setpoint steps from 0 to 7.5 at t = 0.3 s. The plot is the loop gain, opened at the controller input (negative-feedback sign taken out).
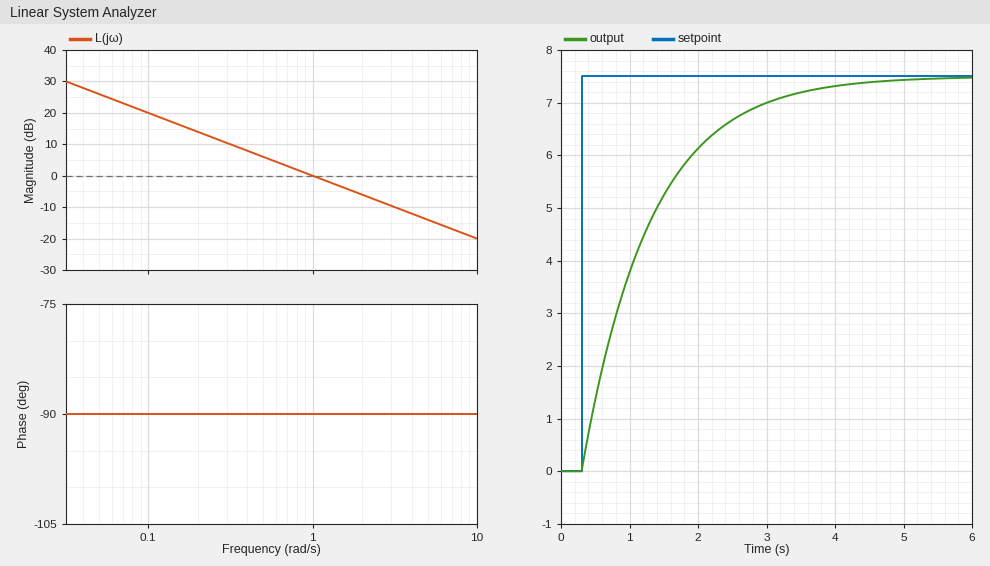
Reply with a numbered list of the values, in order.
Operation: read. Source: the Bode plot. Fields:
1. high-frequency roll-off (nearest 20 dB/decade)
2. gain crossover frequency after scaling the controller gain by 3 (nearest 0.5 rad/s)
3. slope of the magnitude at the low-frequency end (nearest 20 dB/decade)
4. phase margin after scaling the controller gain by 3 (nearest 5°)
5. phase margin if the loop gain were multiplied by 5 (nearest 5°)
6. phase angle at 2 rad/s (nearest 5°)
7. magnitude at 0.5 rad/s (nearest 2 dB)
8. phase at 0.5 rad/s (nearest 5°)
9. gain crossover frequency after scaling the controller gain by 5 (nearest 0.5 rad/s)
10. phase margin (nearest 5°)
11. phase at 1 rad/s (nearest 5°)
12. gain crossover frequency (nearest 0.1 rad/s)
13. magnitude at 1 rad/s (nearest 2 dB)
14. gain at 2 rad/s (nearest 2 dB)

1. -20 dB/decade
2. 3.0 rad/s
3. -20 dB/decade
4. 90°
5. 90°
6. -90°
7. 6 dB
8. -90°
9. 5.0 rad/s
10. 90°
11. -90°
12. 1.0 rad/s
13. 0 dB
14. -6 dB
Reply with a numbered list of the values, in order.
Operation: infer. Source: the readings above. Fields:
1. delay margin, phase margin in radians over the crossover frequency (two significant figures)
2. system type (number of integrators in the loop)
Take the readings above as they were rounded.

1. 1.6 s
2. 1
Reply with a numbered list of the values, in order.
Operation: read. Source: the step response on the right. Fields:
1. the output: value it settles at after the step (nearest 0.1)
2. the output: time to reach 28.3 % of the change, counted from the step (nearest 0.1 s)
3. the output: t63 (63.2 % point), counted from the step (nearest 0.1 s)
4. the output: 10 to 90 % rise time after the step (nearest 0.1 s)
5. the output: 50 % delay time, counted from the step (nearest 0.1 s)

1. 7.5
2. 0.3 s
3. 1.0 s
4. 2.2 s
5. 0.7 s
